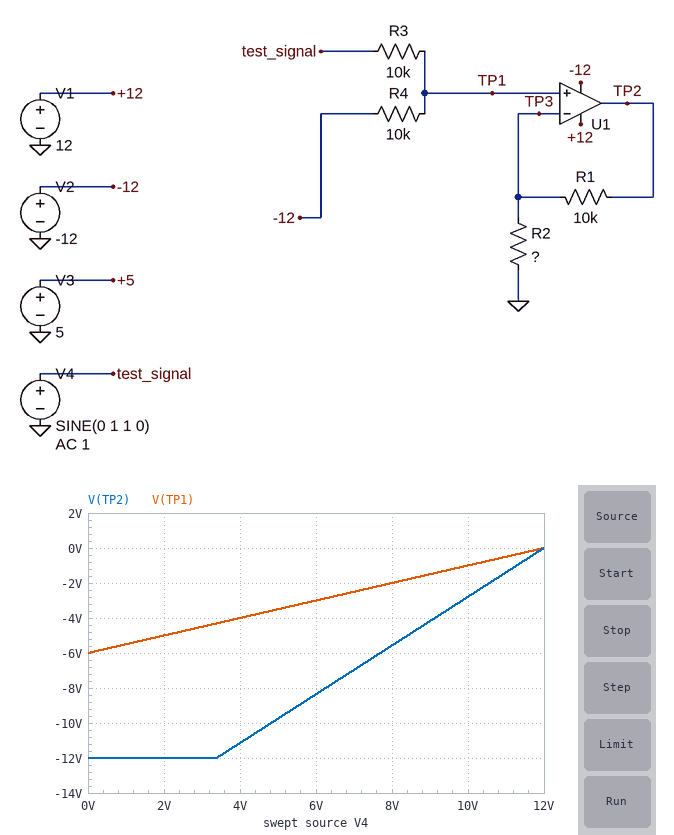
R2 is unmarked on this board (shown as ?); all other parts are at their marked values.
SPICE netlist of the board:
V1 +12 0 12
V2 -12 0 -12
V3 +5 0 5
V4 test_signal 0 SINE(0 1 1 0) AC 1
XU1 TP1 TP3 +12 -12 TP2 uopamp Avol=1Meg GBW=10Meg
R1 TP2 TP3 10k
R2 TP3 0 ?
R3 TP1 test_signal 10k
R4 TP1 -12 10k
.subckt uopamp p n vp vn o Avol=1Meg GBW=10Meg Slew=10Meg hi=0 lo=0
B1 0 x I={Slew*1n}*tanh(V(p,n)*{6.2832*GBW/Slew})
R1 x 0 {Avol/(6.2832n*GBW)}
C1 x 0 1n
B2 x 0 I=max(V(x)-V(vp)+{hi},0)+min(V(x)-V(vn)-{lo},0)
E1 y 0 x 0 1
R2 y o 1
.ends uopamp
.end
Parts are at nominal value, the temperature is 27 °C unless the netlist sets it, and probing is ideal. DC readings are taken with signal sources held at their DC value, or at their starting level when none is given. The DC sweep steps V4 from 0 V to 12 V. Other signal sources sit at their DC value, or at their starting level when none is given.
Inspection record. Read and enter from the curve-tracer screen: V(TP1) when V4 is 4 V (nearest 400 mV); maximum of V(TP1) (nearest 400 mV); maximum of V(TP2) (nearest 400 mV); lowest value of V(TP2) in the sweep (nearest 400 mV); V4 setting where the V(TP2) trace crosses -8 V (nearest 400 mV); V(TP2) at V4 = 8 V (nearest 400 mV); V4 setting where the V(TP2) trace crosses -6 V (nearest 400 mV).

-4.0 V
0 V
0 V
-12.0 V
6.4 V
-5.6 V
7.6 V
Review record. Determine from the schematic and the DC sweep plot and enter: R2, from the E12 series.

5.6 kΩ
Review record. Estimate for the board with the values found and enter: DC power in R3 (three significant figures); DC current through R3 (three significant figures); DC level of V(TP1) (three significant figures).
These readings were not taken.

3.60 mW
600 µA
-6.00 V
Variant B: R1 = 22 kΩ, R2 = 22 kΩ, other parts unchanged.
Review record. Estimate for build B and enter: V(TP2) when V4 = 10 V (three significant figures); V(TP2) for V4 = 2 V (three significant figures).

-2.00 V
-10.0 V
